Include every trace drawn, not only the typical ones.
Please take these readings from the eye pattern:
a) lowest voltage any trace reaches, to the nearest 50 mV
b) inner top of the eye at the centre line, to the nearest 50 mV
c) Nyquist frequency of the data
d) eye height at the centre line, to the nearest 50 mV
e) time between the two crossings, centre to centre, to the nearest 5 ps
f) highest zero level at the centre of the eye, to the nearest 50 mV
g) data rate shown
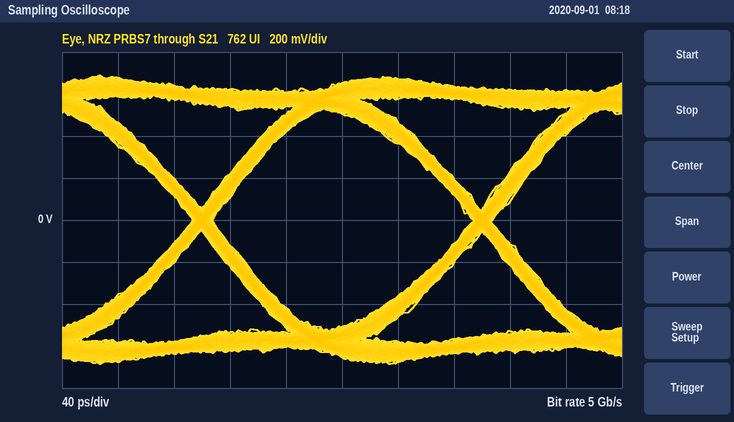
-700 mV
500 mV
2.5 GHz
1.00 V
200 ps
-500 mV
5 Gb/s
